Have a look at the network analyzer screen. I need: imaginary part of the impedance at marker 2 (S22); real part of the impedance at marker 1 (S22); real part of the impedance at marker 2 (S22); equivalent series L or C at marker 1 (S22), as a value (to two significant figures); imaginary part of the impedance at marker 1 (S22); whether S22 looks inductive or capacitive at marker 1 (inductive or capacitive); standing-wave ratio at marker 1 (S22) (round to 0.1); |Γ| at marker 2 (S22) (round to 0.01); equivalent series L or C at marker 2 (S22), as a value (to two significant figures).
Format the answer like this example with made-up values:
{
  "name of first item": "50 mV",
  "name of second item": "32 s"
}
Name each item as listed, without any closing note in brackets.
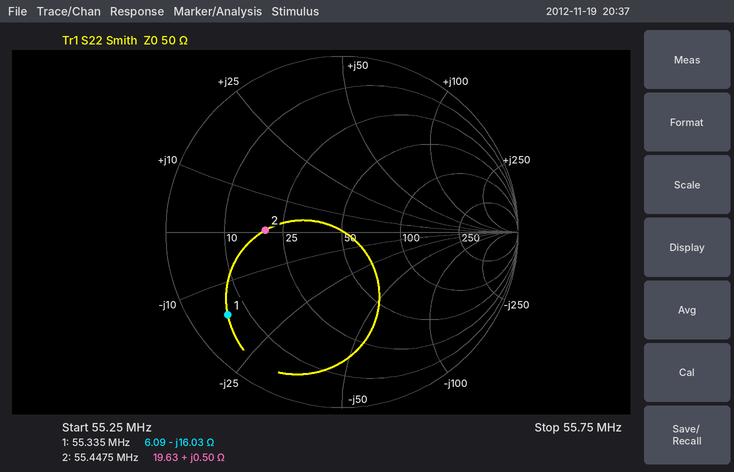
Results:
{
  "imaginary part of the impedance at marker 2": "+0.50 Ω",
  "real part of the impedance at marker 1": "6.09 Ω",
  "real part of the impedance at marker 2": "19.63 Ω",
  "equivalent series L or C at marker 1 (S22), as a value": "180 pF",
  "imaginary part of the impedance at marker 1": "-16.03 Ω",
  "whether S22 looks inductive or capacitive at marker 1": "capacitive",
  "standing-wave ratio at marker 1 (S22)": "9.1",
  "|Γ| at marker 2 (S22)": "0.44",
  "equivalent series L or C at marker 2 (S22), as a value": "1.4 nH"
}
